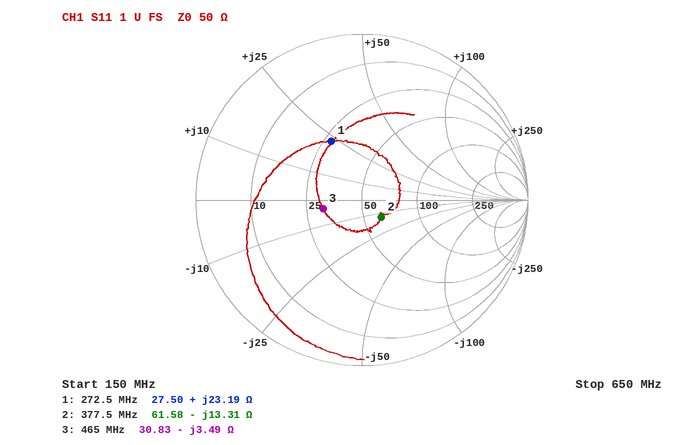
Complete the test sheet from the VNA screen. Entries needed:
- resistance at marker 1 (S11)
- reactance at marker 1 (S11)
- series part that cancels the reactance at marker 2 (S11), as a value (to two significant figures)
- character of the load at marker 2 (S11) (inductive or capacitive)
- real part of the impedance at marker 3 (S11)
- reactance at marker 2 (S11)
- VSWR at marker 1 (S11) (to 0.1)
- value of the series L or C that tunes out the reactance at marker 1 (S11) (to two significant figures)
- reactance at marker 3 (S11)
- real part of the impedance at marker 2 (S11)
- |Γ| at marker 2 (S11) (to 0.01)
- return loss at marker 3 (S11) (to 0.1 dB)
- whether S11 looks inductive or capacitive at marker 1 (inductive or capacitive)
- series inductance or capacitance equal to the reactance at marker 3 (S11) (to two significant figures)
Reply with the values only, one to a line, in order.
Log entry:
27.50 Ω
+23.19 Ω
5.6 nH
capacitive
30.83 Ω
-13.31 Ω
2.3
25 pF
-3.49 Ω
61.58 Ω
0.16
12.4 dB
inductive
98 pF
